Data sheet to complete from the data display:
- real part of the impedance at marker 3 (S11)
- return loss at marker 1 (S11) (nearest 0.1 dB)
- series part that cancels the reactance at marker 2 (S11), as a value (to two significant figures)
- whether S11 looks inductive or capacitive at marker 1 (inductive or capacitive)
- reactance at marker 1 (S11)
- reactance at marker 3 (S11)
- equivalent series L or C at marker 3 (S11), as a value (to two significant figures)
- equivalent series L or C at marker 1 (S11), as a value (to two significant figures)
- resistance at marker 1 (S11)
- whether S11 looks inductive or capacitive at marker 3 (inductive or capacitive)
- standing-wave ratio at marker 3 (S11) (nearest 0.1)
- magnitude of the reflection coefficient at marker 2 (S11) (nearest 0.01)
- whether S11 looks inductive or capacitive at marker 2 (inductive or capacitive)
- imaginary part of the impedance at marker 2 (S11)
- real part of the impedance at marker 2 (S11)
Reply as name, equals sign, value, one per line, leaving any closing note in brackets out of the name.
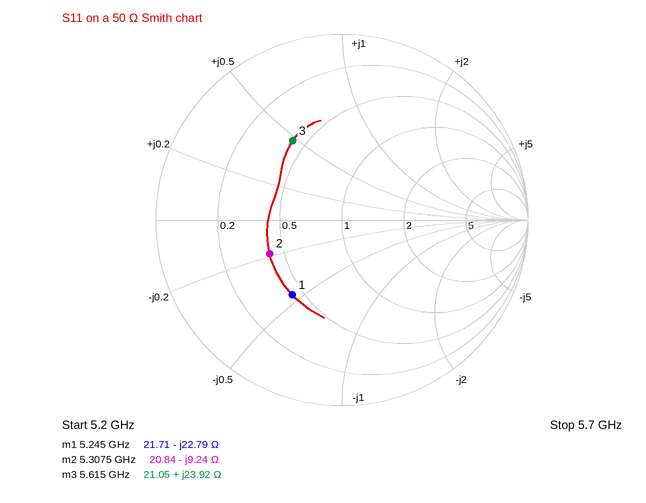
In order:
real part of the impedance at marker 3 = 21.05 Ω
return loss at marker 1 (S11) = 6.3 dB
series part that cancels the reactance at marker 2 (S11), as a value = 280 pH
whether S11 looks inductive or capacitive at marker 1 = capacitive
reactance at marker 1 = -22.79 Ω
reactance at marker 3 = +23.92 Ω
equivalent series L or C at marker 3 (S11), as a value = 680 pH
equivalent series L or C at marker 1 (S11), as a value = 1.3 pF
resistance at marker 1 = 21.71 Ω
whether S11 looks inductive or capacitive at marker 3 = inductive
standing-wave ratio at marker 3 (S11) = 3.0
magnitude of the reflection coefficient at marker 2 (S11) = 0.43
whether S11 looks inductive or capacitive at marker 2 = capacitive
imaginary part of the impedance at marker 2 = -9.24 Ω
real part of the impedance at marker 2 = 20.84 Ω
